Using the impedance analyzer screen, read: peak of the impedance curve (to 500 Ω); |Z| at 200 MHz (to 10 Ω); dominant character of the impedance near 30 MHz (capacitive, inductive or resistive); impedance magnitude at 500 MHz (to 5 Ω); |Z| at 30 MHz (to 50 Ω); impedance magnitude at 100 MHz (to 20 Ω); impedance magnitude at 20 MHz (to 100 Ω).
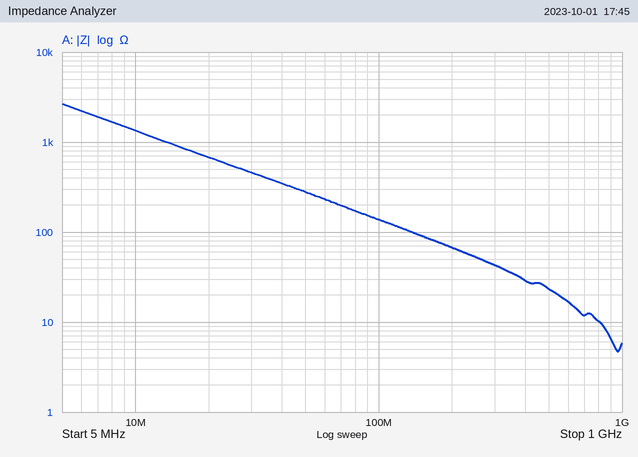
2.5 kΩ
70 Ω
capacitive
25 Ω
450 Ω
140 Ω
700 Ω
